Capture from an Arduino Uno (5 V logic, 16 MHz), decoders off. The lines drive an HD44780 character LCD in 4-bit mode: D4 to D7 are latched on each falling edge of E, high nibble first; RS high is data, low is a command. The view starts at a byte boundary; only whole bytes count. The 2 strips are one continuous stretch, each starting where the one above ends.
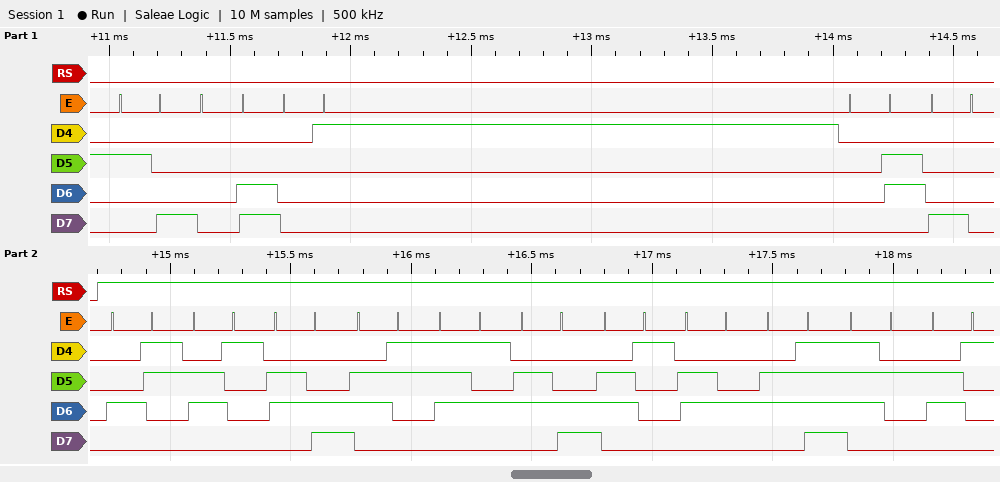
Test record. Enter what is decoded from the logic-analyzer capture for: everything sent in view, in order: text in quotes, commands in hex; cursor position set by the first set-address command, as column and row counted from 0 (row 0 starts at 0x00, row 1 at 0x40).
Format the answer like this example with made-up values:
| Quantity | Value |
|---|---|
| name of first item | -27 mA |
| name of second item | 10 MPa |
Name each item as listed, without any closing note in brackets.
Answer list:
| Quantity | Value |
|---|---|
| everything sent in view, in order: text in quotes, commands in hex | 0x28 0x0C 0x01 0x06 0x80 "Calculadora" |
| cursor position set by the first set-address command, as column and row counted from 0 | column 0, row 0 |
